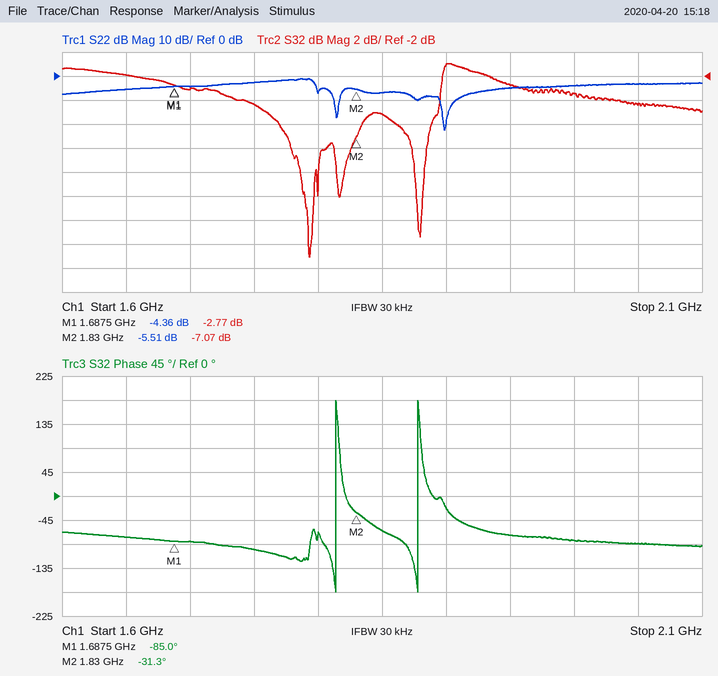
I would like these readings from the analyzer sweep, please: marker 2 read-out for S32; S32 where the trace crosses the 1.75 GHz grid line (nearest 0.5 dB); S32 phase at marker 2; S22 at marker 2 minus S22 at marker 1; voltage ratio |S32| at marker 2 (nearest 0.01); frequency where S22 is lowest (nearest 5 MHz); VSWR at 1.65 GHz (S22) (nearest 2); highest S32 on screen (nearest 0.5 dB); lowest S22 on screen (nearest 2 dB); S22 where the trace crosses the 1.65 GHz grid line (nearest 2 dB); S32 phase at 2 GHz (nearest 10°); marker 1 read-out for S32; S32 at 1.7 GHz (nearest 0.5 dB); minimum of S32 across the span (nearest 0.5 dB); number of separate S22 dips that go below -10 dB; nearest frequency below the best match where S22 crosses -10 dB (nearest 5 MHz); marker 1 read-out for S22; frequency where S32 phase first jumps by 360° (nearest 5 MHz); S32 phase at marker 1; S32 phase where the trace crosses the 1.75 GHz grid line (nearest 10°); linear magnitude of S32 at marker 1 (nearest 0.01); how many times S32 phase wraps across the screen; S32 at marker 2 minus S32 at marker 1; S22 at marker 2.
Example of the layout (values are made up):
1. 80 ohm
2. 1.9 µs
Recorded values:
1. -7.07 dB
2. -4.5 dB
3. -31.3°
4. -1.15 dB
5. 0.44
6. 1.900 GHz
7. 4
8. -1.0 dB
9. -22 dB
10. -6 dB
11. -80°
12. -2.77 dB
13. -3.0 dB
14. -17.0 dB
15. 2
16. 1.895 GHz
17. -4.36 dB
18. 1.815 GHz
19. -85.0°
20. -100°
21. 0.73
22. 2
23. -4.30 dB
24. -5.51 dB
